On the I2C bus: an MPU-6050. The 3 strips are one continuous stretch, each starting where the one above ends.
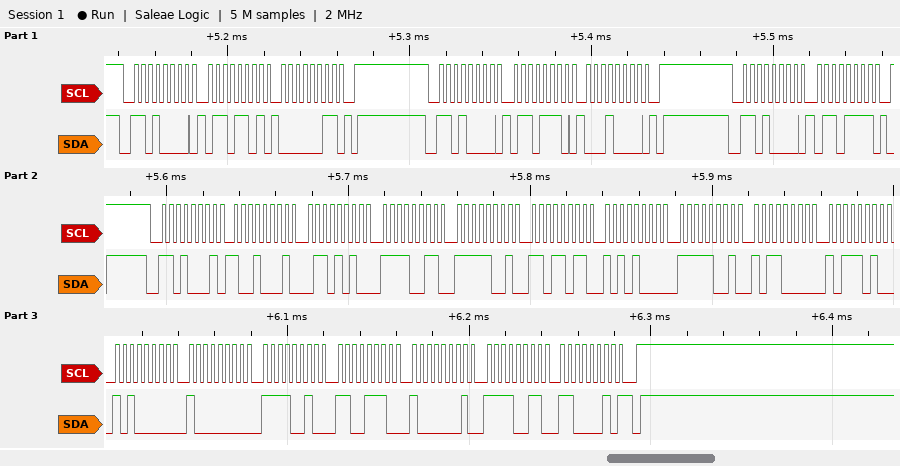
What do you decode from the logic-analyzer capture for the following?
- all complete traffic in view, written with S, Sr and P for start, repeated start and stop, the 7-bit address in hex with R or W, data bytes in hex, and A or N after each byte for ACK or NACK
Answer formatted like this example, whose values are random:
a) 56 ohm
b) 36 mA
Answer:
a) S 68W A 6D A 03 A P S 68W A 6E A 10 A P S 68W A 6F A P S 68R A 91 A 6A A F3 A F9 A DB A A8 A F9 A B0 A BA A A0 A 80 A F2 A CE A 81 A F3 A C2 N P
